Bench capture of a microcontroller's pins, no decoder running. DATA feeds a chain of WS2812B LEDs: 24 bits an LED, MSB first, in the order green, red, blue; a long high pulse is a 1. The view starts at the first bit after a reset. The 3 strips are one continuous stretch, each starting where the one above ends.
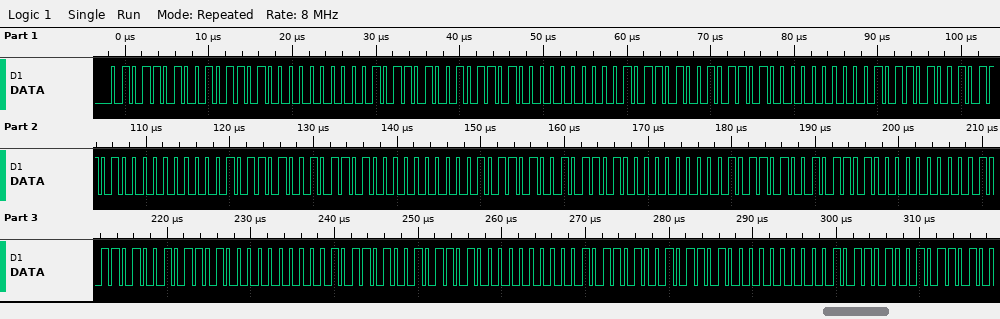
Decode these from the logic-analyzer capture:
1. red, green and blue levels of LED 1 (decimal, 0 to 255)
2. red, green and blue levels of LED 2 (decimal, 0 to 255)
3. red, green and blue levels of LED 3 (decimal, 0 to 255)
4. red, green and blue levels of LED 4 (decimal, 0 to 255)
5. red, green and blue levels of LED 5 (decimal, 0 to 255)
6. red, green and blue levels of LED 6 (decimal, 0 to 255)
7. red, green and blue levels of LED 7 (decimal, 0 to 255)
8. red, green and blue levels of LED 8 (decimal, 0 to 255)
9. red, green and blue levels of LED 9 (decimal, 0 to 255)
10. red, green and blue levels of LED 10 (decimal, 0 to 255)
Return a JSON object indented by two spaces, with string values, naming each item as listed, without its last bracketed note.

{
  "red, green and blue levels of LED 1": "90, 90, 0",
  "red, green and blue levels of LED 2": "90, 90, 0",
  "red, green and blue levels of LED 3": "90, 90, 0",
  "red, green and blue levels of LED 4": "90, 90, 0",
  "red, green and blue levels of LED 5": "90, 90, 0",
  "red, green and blue levels of LED 6": "90, 90, 0",
  "red, green and blue levels of LED 7": "90, 90, 0",
  "red, green and blue levels of LED 8": "90, 90, 0",
  "red, green and blue levels of LED 9": "90, 90, 0",
  "red, green and blue levels of LED 10": "90, 90, 0"
}
